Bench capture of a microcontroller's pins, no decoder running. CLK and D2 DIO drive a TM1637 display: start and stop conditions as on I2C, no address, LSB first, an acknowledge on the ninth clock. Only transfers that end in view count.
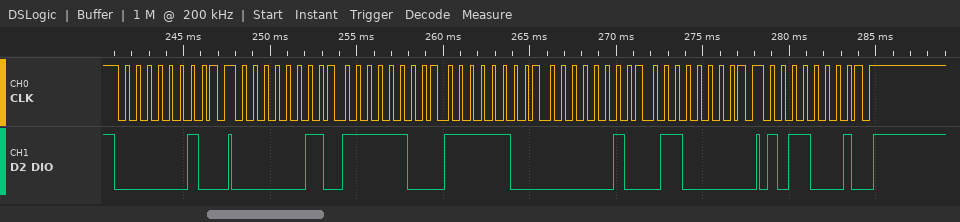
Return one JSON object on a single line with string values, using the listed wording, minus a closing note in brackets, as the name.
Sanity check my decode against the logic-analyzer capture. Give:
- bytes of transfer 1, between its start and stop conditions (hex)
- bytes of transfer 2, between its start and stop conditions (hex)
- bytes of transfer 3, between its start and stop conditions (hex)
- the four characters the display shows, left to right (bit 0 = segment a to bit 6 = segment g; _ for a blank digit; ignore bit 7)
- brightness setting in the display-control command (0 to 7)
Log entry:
{"bytes of transfer 1, between its start and stop conditions": "40", "bytes of transfer 2, between its start and stop conditions": "C0 3F 3F 40 06", "bytes of transfer 3, between its start and stop conditions": "8D", "the four characters the display shows, left to right": "00-1", "brightness setting in the display-control command": "5"}
